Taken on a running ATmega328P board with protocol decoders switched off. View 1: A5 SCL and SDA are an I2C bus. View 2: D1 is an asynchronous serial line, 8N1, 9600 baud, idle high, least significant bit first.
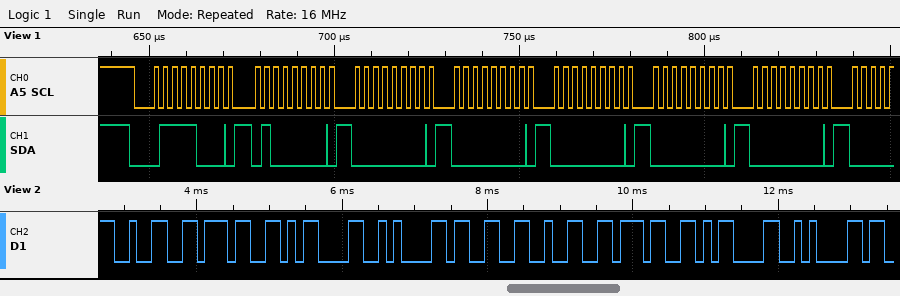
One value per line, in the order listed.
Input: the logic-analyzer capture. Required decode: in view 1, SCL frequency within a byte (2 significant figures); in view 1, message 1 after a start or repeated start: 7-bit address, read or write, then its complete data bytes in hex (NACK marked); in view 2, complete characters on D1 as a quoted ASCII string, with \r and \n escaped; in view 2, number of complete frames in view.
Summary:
400 kHz
0x3C write: 40 00 00 00 00 00
"27\r\n327\r\n"
9
